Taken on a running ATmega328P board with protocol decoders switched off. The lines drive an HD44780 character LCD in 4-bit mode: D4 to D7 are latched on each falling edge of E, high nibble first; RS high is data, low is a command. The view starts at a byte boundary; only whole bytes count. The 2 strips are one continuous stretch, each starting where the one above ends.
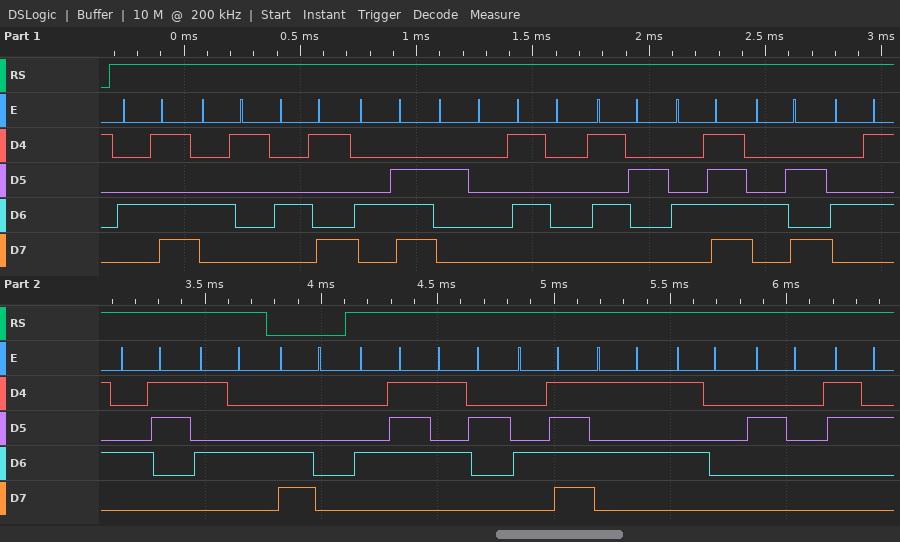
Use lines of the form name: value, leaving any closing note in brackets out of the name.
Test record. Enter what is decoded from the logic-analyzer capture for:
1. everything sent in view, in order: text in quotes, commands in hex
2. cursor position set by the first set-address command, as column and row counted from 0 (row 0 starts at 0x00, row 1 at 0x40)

everything sent in view, in order: text in quotes, commands in hex: "MAIN PROJECT" 0xC0 "GROUP 2"
cursor position set by the first set-address command, as column and row counted from 0: column 0, row 1
